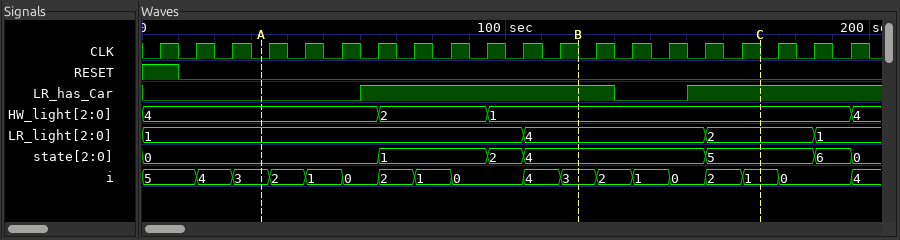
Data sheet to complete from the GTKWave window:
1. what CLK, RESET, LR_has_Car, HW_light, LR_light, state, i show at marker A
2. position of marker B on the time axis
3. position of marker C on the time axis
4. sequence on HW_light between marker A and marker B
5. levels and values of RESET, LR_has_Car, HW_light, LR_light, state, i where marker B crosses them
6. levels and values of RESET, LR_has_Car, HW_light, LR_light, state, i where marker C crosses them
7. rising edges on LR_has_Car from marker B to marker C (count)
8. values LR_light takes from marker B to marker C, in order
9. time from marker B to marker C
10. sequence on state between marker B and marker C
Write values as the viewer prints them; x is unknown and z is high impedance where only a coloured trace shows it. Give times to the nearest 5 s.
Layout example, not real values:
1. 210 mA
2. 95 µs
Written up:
1. CLK=0, RESET=0, LR_has_Car=0, HW_light=4, LR_light=1, state=0, i=3
2. 120 s
3. 170 s
4. 4, 2, 1
5. RESET=0, LR_has_Car=1, HW_light=1, LR_light=4, state=4, i=3
6. RESET=0, LR_has_Car=1, HW_light=1, LR_light=2, state=5, i=1
7. 1
8. 4, 2
9. 50 s
10. 4, 5
